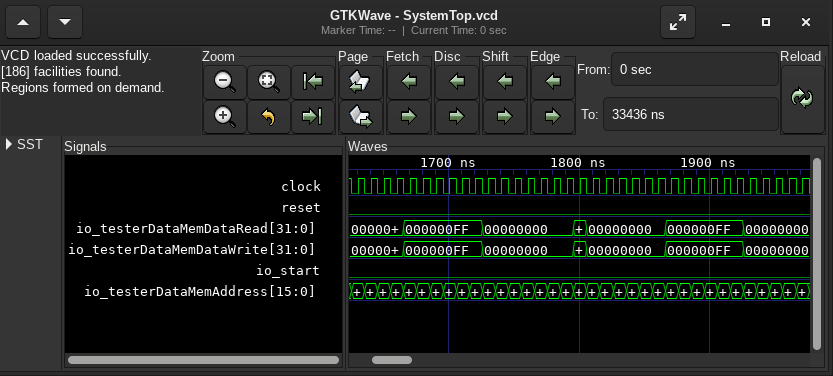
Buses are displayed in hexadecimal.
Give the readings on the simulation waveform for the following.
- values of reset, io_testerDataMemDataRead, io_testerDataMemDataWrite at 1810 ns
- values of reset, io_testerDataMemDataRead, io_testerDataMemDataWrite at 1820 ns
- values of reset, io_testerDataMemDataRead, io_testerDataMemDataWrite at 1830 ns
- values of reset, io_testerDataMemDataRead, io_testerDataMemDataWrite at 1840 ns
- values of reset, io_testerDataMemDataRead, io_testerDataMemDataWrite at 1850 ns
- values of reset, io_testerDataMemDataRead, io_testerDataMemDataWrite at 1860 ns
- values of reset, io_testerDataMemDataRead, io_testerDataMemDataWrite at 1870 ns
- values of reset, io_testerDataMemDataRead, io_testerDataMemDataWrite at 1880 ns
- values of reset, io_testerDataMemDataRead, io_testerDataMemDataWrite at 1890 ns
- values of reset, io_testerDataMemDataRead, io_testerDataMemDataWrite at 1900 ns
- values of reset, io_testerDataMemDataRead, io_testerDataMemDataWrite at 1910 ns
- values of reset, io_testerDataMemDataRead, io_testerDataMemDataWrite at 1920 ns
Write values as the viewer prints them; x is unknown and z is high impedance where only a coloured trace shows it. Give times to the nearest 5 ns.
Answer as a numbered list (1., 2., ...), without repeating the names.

1. reset=0, io_testerDataMemDataRead=00000000, io_testerDataMemDataWrite=00000000
2. reset=0, io_testerDataMemDataRead=00000000, io_testerDataMemDataWrite=00000000
3. reset=0, io_testerDataMemDataRead=00000000, io_testerDataMemDataWrite=00000000
4. reset=0, io_testerDataMemDataRead=00000000, io_testerDataMemDataWrite=00000000
5. reset=0, io_testerDataMemDataRead=00000000, io_testerDataMemDataWrite=00000000
6. reset=0, io_testerDataMemDataRead=00000000, io_testerDataMemDataWrite=00000000
7. reset=0, io_testerDataMemDataRead=000000FF, io_testerDataMemDataWrite=000000FF
8. reset=0, io_testerDataMemDataRead=000000FF, io_testerDataMemDataWrite=000000FF
9. reset=0, io_testerDataMemDataRead=000000FF, io_testerDataMemDataWrite=000000FF
10. reset=0, io_testerDataMemDataRead=000000FF, io_testerDataMemDataWrite=000000FF
11. reset=0, io_testerDataMemDataRead=000000FF, io_testerDataMemDataWrite=000000FF
12. reset=0, io_testerDataMemDataRead=000000FF, io_testerDataMemDataWrite=000000FF
